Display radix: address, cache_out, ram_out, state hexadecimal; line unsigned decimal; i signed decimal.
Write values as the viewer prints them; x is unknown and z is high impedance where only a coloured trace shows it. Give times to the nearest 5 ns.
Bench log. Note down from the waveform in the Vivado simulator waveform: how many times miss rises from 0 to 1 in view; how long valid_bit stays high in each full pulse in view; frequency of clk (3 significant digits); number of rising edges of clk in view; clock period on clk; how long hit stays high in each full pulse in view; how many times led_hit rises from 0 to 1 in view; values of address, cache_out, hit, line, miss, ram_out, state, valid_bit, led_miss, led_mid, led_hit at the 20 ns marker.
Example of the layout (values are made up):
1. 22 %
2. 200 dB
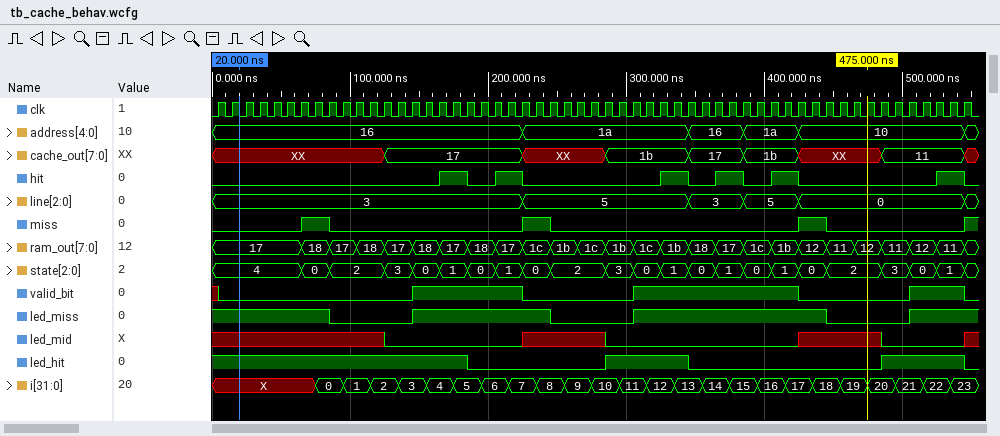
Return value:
1. 4
2. 80 ns, 120 ns, 40 ns
3. 100 MHz
4. 55
5. 10 ns
6. 20 ns, 20 ns, 20 ns, 20 ns, 20 ns, 20 ns
7. 2
8. address=16, cache_out=XX, hit=0, line=3, miss=0, ram_out=17, state=4, valid_bit=0, led_miss=1, led_mid=x, led_hit=1
